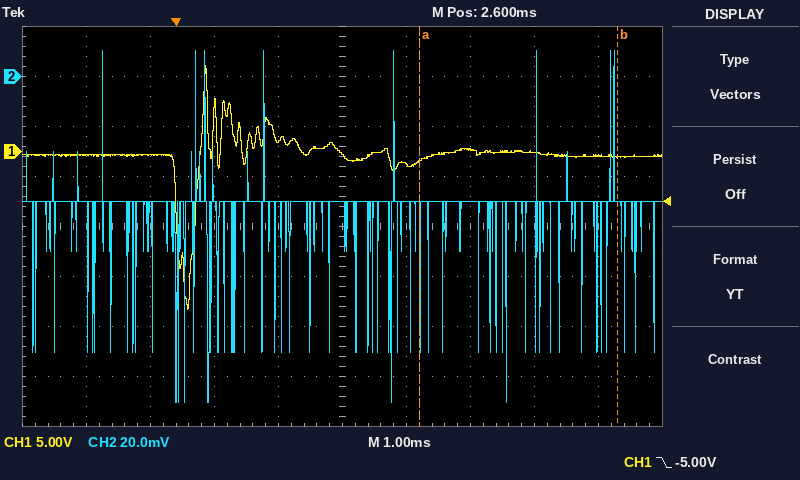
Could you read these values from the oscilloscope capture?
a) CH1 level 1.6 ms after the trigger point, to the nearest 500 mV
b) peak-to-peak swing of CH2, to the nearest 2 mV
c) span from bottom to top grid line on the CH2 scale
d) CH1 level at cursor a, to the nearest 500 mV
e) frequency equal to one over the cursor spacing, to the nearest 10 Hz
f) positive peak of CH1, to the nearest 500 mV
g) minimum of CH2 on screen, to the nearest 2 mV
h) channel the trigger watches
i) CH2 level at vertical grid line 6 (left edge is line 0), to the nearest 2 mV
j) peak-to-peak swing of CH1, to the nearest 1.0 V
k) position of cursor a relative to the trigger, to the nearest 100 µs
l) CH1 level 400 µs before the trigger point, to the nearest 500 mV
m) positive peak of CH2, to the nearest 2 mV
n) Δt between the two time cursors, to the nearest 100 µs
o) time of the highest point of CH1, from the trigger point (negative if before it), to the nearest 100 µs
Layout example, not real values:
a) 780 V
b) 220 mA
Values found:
a) 1.0 V
b) 140 mV
c) 160 mV
d) -1.0 V
e) 320 Hz
f) 8.5 V
g) -130 mV
h) CH1
i) -50 mV
j) 24.0 V
k) +3.8 ms
l) -500 mV
m) 10 mV
n) 3.1 ms
o) +500 µs
